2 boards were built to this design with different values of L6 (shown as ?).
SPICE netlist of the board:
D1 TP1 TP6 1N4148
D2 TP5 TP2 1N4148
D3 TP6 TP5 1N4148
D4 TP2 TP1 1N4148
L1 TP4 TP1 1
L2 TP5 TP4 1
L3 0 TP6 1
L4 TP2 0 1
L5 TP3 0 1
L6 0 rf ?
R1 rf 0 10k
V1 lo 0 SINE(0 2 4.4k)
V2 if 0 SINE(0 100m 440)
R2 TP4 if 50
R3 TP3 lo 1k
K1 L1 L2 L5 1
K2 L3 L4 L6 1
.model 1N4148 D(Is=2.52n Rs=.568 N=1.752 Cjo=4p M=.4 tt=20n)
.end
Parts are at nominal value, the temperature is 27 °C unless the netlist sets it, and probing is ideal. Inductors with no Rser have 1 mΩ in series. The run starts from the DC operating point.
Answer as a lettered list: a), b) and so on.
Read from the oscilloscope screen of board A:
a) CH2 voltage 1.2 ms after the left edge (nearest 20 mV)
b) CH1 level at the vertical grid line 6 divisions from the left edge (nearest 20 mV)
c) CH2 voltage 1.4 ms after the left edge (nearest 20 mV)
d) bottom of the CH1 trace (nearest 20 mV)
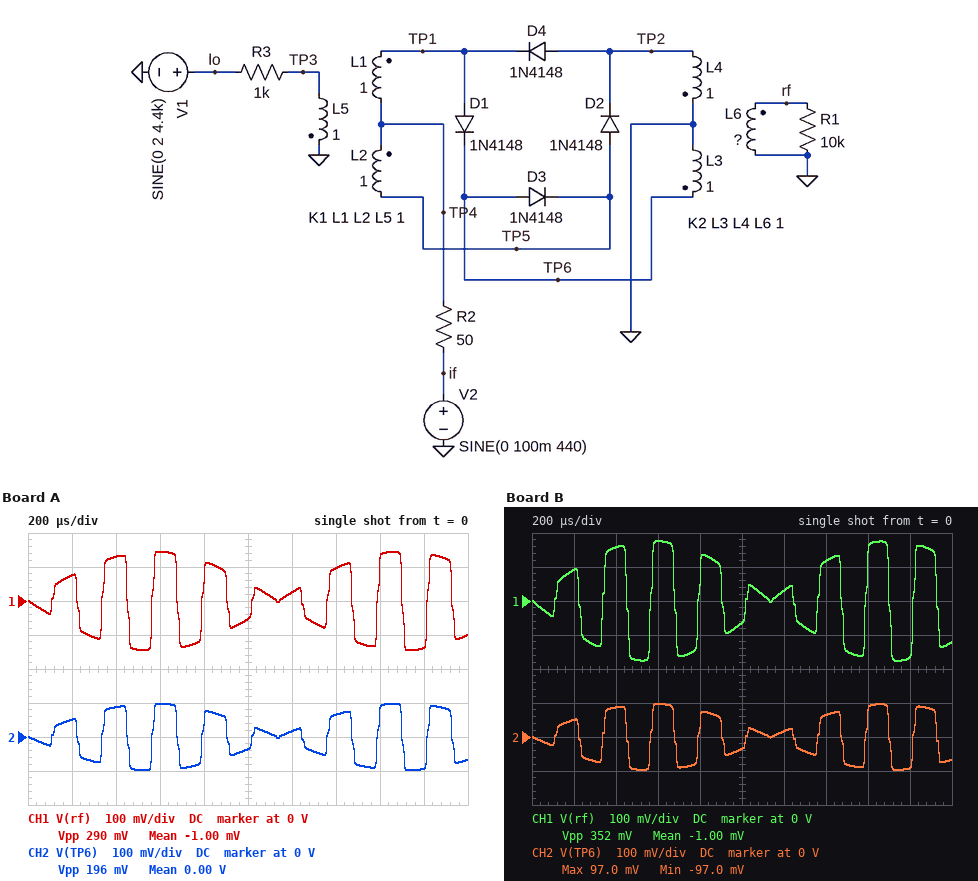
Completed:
a) 20 mV
b) 20 mV
c) 60 mV
d) -140 mV
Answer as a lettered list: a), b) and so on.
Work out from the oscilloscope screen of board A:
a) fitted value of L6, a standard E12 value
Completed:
a) 2.2 H
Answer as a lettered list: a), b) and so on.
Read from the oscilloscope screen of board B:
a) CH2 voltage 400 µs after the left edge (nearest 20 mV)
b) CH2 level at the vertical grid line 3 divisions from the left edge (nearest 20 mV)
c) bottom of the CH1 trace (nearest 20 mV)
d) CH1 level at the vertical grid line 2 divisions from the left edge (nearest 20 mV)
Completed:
a) 80 mV
b) 100 mV
c) -180 mV
d) 160 mV
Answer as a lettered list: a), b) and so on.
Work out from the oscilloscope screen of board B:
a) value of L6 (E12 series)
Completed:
a) 3.3 H
